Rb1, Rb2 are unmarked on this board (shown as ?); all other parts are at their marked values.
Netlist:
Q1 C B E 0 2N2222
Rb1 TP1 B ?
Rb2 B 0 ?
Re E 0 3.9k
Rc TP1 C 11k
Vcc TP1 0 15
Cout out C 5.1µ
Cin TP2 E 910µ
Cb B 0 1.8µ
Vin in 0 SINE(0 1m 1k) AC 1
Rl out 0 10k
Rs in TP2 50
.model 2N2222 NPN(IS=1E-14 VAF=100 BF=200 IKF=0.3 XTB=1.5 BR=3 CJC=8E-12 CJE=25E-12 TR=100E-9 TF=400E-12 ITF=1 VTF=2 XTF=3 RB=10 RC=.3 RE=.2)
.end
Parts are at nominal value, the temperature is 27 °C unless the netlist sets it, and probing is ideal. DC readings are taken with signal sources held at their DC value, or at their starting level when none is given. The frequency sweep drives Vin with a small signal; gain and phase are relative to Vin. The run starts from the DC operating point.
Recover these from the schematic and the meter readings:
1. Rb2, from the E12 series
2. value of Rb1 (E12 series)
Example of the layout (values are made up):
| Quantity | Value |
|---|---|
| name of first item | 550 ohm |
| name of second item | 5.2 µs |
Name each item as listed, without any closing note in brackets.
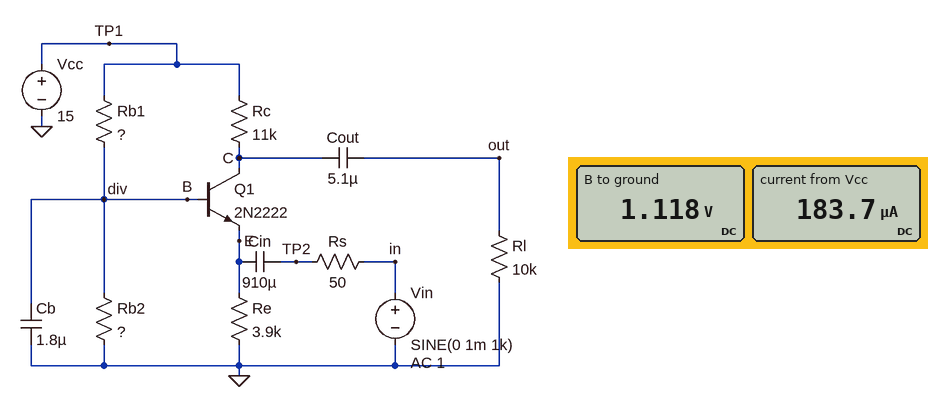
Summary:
| Quantity | Value |
|---|---|
| Rb2, from the E12 series | 22 kΩ |
| value of Rb1 | 270 kΩ |
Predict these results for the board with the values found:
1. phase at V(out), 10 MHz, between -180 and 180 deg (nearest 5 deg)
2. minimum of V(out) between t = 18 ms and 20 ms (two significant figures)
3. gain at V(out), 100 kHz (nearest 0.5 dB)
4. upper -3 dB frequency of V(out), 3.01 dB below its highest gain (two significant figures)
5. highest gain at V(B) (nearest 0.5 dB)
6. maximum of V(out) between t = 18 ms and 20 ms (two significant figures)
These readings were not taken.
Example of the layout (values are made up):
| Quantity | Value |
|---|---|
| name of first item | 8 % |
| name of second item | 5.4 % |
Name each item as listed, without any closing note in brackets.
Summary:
| Quantity | Value |
|---|---|
| phase at V(out), 10 MHz, between -180 and 180 deg | -55 deg |
| minimum of V(out) between t = 18 ms and 20 ms | -21 mV |
| gain at V(out), 100 kHz | 26.5 dB |
| upper -3 dB frequency of V(out), 3.01 dB below its highest gain | 9.3 MHz |
| highest gain at V(B) | -12.5 dB |
| maximum of V(out) between t = 18 ms and 20 ms | 21 mV |
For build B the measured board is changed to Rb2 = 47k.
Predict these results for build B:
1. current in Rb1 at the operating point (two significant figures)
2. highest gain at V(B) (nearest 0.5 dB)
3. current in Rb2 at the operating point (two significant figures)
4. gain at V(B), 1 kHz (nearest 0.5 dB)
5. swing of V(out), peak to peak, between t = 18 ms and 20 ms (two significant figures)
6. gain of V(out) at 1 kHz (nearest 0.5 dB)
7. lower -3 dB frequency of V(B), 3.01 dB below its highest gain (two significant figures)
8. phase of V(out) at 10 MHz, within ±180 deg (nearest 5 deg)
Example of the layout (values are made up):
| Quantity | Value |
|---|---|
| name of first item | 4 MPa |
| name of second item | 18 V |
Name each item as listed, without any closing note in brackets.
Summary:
| Quantity | Value |
|---|---|
| current in Rb1 at the operating point | 48 µA |
| highest gain at V(B) | -6.5 dB |
| current in Rb2 at the operating point | 46 µA |
| gain at V(B), 1 kHz | -49.0 dB |
| swing of V(out), peak to peak, between t = 18 ms and 20 ms | 88 mV |
| gain of V(out) at 1 kHz | 33.0 dB |
| lower -3 dB frequency of V(B), 3.01 dB below its highest gain | 440 mHz |
| phase of V(out) at 10 MHz, within ±180 deg | -55 deg |
